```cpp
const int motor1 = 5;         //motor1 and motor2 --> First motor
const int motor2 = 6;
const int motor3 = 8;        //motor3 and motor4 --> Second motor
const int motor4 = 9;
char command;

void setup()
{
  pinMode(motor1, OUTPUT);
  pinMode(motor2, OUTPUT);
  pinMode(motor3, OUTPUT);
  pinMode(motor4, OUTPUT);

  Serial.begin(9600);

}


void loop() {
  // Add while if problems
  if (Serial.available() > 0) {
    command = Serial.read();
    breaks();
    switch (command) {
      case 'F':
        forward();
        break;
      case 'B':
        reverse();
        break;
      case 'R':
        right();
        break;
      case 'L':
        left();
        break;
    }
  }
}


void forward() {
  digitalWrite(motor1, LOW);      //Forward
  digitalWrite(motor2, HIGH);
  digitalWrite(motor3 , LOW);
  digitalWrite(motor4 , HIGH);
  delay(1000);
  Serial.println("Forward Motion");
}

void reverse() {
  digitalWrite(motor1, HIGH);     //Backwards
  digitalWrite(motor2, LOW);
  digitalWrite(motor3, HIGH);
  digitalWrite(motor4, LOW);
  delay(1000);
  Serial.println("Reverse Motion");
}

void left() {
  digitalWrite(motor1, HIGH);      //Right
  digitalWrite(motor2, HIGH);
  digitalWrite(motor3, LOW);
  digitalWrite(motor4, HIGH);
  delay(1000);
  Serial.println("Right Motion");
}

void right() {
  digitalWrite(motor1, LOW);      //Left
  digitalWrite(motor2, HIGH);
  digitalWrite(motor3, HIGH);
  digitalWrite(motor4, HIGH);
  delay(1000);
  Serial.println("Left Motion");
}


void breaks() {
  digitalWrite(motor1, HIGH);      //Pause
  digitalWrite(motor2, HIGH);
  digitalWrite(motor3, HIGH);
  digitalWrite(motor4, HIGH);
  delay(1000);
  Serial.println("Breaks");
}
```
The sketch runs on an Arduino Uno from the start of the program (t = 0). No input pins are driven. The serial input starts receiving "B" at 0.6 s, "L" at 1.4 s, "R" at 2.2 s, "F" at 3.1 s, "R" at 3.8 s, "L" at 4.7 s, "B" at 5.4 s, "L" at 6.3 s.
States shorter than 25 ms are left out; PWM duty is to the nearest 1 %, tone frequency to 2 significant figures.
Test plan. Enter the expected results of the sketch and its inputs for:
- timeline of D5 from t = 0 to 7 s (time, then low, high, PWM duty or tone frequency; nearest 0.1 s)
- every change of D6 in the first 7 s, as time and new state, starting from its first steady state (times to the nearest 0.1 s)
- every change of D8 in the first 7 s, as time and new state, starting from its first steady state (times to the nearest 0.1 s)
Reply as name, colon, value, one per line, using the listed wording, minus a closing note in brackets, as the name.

timeline of D5 from t = 0 to 7 s: 0 s low; 0.6 s high; 5.6 s low; 6.6 s high
every change of D6 in the first 7 s, as time and new state, starting from its first steady state: 0 s low; 0.6 s high; 1.6 s low; 2.6 s high
every change of D8 in the first 7 s, as time and new state, starting from its first steady state: 0 s low; 0.6 s high; 3.6 s low; 4.6 s high
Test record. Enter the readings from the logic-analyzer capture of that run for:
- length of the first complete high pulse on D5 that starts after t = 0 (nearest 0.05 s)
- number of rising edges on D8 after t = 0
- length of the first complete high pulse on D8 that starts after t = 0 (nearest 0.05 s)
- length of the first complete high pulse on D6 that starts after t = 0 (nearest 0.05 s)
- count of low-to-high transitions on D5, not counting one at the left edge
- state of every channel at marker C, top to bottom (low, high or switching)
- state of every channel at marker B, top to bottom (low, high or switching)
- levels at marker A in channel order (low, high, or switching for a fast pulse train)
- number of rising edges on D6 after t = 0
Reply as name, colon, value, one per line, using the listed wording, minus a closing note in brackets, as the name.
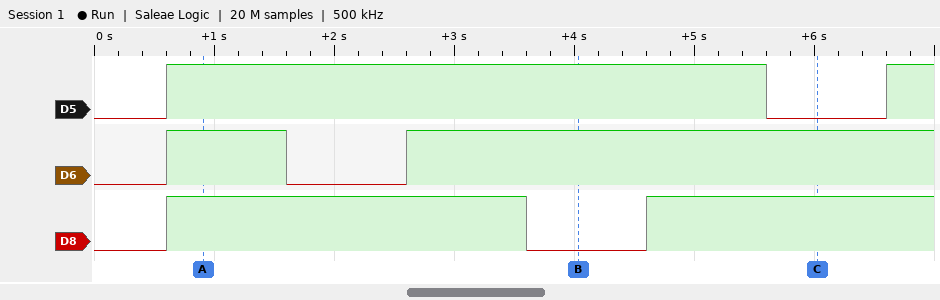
length of the first complete high pulse on D5 that starts after t = 0: 5.00 s
number of rising edges on D8 after t = 0: 2
length of the first complete high pulse on D8 that starts after t = 0: 3.00 s
length of the first complete high pulse on D6 that starts after t = 0: 1.00 s
count of low-to-high transitions on D5, not counting one at the left edge: 2
state of every channel at marker C, top to bottom: D5 low, D6 high, D8 high
state of every channel at marker B, top to bottom: D5 high, D6 high, D8 low
levels at marker A in channel order: D5 high, D6 high, D8 high
number of rising edges on D6 after t = 0: 2
